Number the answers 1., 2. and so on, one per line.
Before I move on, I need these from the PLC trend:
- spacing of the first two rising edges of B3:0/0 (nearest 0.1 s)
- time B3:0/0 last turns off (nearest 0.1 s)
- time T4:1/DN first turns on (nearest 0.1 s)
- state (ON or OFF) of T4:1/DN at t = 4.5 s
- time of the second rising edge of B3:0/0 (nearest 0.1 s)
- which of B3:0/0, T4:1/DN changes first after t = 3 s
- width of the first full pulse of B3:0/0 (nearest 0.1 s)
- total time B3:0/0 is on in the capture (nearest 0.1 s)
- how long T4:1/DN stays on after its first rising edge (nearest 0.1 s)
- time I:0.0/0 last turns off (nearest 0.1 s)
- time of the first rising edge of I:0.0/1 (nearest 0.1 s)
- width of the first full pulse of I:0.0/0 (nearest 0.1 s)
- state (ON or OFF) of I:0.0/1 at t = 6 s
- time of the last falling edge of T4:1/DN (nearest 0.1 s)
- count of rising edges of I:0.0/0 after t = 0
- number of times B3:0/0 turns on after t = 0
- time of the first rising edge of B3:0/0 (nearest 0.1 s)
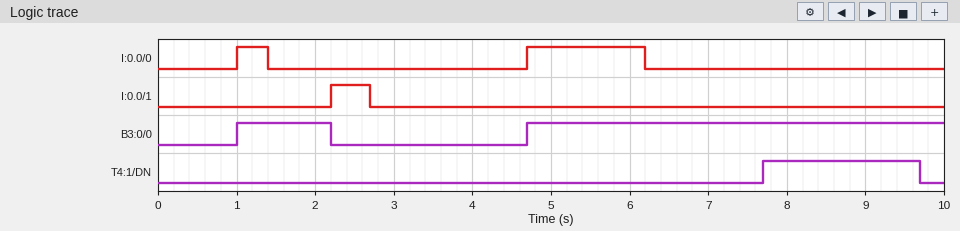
1. 3.7 s
2. 2.2 s
3. 7.7 s
4. OFF
5. 4.7 s
6. B3:0/0
7. 1.2 s
8. 6.5 s
9. 2.0 s
10. 6.2 s
11. 2.2 s
12. 0.4 s
13. OFF
14. 9.7 s
15. 2
16. 2
17. 1.0 s
